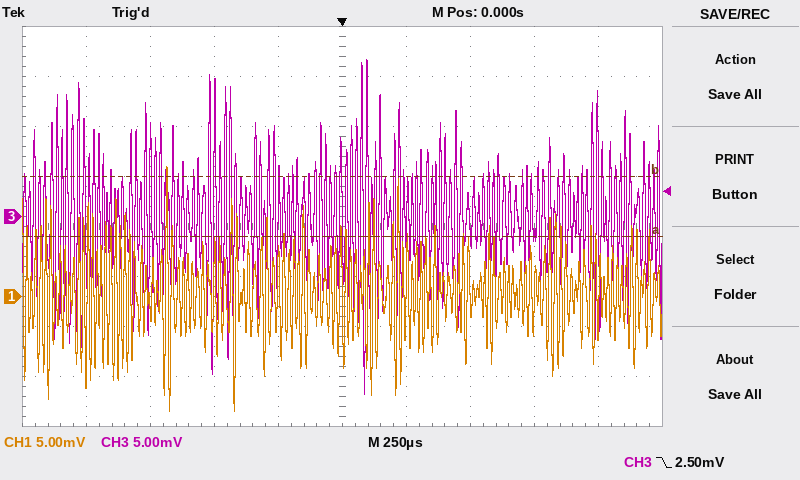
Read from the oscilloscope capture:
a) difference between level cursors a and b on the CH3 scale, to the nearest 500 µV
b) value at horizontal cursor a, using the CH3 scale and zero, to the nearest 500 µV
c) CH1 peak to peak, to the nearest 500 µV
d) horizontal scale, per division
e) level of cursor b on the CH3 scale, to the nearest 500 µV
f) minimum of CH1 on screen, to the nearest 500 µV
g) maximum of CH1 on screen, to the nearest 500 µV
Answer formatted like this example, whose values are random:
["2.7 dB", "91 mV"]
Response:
["6.0 mV", "-2.0 mV", "24.5 mV", "250 µs", "4.0 mV", "-11.5 mV", "13.0 mV"]
